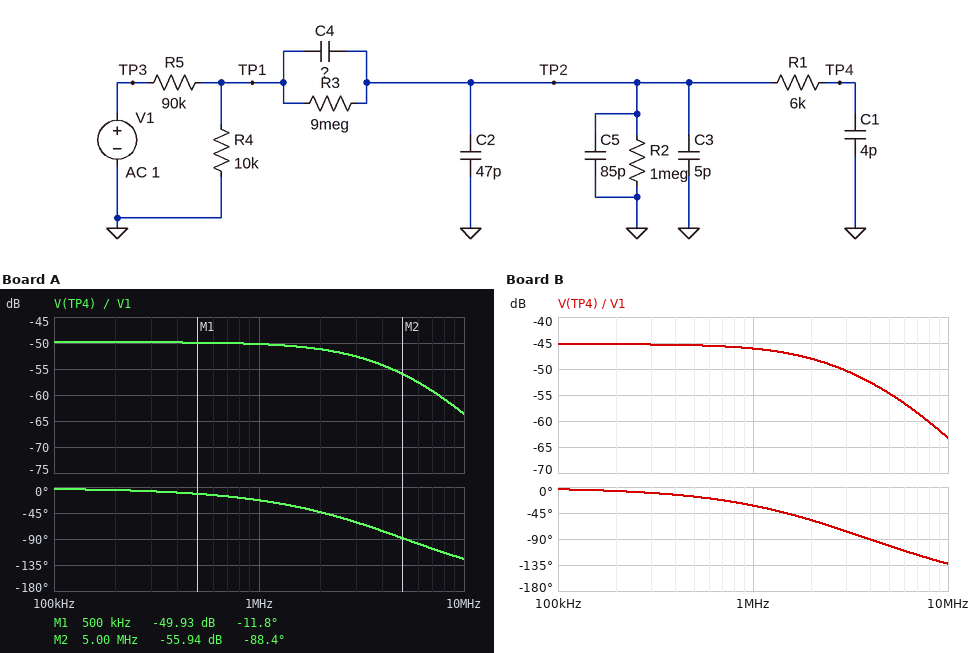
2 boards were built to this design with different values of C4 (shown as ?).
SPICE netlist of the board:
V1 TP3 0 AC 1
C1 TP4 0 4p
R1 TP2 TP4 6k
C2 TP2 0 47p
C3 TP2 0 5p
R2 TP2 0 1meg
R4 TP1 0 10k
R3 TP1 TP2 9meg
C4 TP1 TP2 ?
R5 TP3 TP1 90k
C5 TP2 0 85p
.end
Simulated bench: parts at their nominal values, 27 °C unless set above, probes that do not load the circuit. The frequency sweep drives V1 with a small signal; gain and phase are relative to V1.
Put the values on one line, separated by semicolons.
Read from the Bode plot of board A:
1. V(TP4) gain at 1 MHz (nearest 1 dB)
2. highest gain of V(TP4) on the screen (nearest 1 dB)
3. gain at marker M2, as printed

-50 dB; -50 dB; -55.94 dB
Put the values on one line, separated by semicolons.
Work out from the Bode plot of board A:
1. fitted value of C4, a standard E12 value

4.7 pF
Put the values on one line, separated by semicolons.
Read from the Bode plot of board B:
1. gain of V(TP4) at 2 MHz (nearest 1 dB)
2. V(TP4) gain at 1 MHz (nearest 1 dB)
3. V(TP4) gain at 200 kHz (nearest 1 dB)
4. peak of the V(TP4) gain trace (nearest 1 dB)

-48 dB; -46 dB; -45 dB; -45 dB
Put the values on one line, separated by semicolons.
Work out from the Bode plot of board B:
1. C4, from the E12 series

8.2 pF
